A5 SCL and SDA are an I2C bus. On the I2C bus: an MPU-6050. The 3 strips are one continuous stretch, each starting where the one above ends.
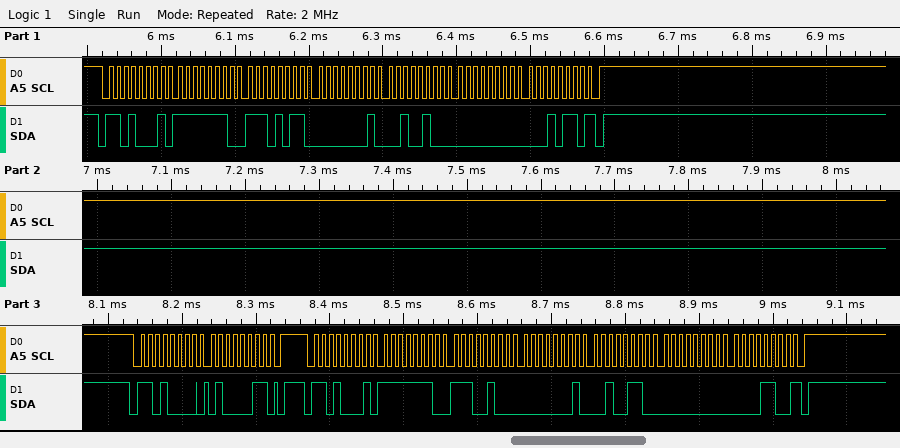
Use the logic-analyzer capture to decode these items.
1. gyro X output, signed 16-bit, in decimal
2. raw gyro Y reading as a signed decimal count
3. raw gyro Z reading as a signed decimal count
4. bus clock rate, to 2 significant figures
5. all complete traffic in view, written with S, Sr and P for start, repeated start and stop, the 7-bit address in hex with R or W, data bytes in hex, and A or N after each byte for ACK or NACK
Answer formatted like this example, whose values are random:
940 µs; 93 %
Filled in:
-284; 294; 12; 100 kHz; S 68R A FE A EB A 01 A 24 A 00 A 16 N P S 68W A 43 A P S 68R A FE A E4 A 01 A 26 A 00 A 0C N P
